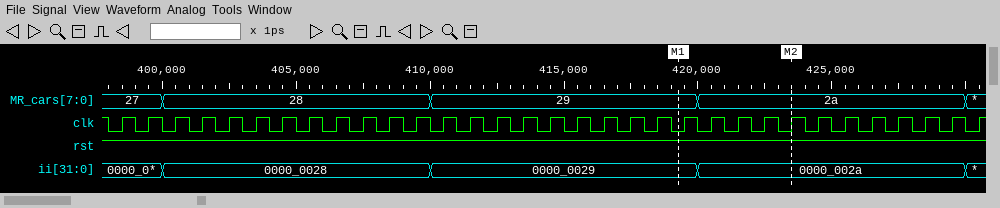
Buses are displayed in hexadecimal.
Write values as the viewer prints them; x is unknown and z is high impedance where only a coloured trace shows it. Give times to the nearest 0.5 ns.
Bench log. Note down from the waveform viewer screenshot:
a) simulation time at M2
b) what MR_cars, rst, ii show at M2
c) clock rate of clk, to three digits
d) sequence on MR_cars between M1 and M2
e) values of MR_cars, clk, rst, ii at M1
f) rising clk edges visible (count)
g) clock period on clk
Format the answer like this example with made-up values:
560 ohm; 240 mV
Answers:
423.5 ns; MR_cars=2a, rst=1, ii=0000_002a; 1.00 GHz; 29, 2a; MR_cars=29, clk=0, rst=1, ii=0000_0029; 33; 1 ns
